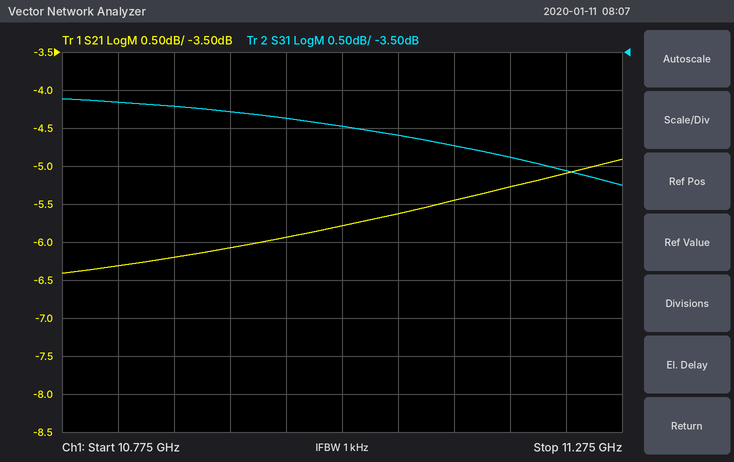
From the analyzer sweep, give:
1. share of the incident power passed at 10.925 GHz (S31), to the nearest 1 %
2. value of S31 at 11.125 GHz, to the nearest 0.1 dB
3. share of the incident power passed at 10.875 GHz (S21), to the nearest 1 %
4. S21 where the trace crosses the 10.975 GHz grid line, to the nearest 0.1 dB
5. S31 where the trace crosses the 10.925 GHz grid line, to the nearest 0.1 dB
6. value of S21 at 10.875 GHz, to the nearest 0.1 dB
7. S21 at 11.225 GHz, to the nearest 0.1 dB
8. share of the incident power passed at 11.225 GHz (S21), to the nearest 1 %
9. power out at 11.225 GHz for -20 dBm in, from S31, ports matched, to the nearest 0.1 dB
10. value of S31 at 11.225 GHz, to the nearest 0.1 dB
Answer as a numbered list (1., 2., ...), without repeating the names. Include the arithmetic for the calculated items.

1. 10^(-4.3/10) ≈ 37 %
2. -4.7 dB
3. 10^(-6.2/10) ≈ 24 %
4. -5.9 dB
5. -4.3 dB
6. -6.2 dB
7. -5.1 dB
8. 10^(-5.1/10) ≈ 31 %
9. -20 dBm + (-5.1 dB) = -25.1 dBm
10. -5.1 dB
